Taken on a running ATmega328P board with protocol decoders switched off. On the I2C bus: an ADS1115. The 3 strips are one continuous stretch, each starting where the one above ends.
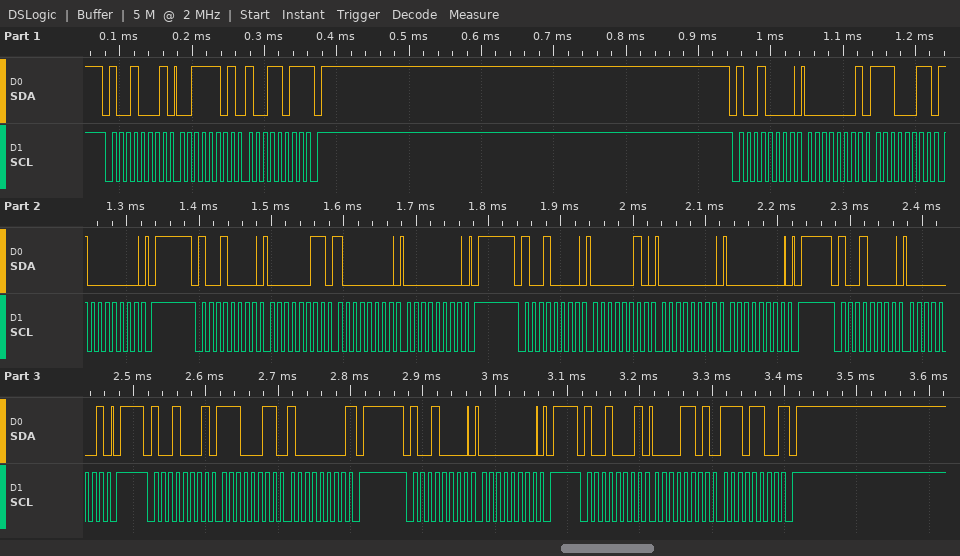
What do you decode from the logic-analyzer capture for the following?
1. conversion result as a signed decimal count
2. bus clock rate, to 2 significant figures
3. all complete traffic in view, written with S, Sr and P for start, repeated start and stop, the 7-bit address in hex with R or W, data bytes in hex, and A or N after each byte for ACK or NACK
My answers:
3564
100 kHz
S 48R A 3D A 9B N P S 48W A 01 A E3 A 80 A P S 48W A 03 A 80 A 00 A P S 48W A 02 A 00 A 00 A P S 48W A 01 A P S 48R A E3 A 80 N P S 48W A 00 A P S 48R A 0D A EC N P
